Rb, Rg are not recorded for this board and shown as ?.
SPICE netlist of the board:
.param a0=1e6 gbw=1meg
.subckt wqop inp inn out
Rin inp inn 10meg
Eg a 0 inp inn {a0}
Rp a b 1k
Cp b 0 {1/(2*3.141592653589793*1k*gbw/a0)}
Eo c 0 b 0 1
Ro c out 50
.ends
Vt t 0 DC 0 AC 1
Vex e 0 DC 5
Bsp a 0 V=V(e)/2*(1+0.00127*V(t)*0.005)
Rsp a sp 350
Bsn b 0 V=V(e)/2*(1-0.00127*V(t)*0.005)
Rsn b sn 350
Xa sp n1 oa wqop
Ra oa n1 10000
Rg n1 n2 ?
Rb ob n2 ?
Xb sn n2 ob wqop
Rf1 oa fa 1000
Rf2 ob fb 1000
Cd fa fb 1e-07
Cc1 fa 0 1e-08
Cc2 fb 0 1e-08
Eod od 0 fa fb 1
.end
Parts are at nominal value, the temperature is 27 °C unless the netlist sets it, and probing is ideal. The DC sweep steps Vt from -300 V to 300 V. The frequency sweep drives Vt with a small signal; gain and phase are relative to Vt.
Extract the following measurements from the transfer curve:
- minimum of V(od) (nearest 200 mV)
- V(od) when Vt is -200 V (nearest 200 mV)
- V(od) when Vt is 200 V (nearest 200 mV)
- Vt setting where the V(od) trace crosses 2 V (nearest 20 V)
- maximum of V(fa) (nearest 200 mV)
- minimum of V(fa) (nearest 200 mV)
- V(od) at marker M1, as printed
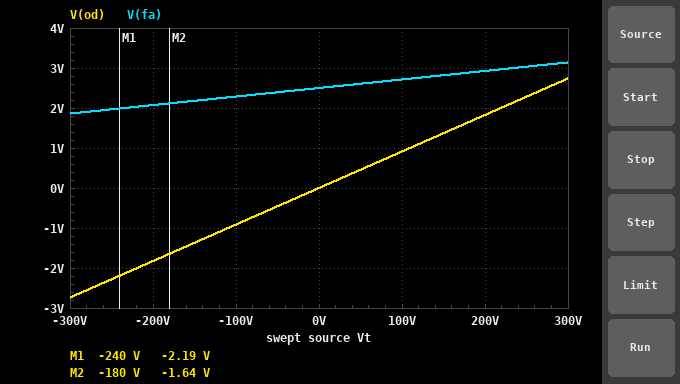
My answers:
-2.8 V
-1.8 V
1.8 V
220 V
3.2 V
1.8 V
-2.19 V
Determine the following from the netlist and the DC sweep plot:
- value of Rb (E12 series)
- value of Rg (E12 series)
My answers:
33 kΩ
150 Ω
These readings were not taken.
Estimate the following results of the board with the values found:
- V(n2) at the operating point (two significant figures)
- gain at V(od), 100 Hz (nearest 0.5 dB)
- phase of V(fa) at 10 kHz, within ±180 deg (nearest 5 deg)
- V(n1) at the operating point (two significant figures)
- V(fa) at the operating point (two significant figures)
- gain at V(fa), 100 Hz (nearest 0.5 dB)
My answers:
2.5 V
-41.0 dB
85 deg
2.5 V
2.5 V
-53.5 dB
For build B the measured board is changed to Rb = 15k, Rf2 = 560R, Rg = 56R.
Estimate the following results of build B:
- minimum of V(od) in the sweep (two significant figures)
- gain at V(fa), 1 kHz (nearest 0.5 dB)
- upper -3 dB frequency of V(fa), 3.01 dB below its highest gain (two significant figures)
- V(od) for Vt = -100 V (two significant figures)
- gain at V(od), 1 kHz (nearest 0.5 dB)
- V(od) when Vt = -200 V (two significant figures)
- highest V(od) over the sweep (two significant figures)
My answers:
-4.3 V
-47.5 dB
1.1 kHz
-1.4 V
-41.0 dB
-2.8 V
4.3 V
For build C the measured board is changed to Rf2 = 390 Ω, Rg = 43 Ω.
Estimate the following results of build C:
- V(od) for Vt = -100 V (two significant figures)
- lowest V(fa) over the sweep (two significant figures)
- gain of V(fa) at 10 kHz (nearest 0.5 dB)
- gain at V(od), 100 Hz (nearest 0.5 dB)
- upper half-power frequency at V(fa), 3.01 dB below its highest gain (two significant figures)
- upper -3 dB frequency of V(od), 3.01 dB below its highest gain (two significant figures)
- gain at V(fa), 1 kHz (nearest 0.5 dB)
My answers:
-3.2 V
280 mV
-58.0 dB
-30.0 dB
1.9 kHz
680 Hz
-42.0 dB
